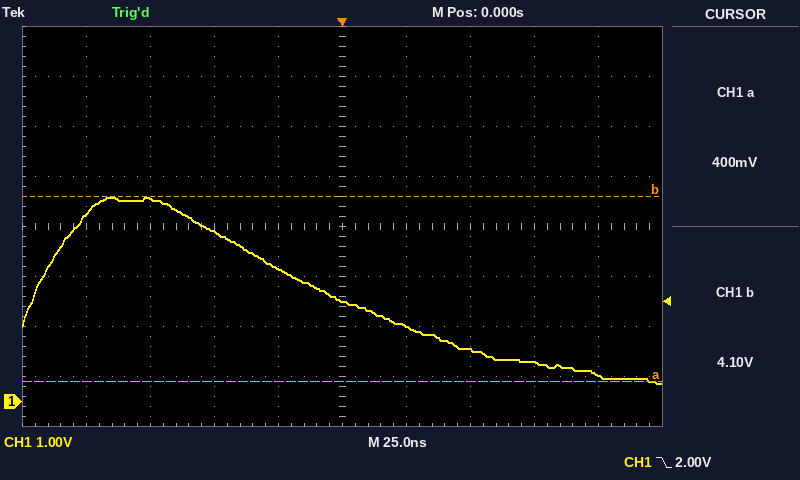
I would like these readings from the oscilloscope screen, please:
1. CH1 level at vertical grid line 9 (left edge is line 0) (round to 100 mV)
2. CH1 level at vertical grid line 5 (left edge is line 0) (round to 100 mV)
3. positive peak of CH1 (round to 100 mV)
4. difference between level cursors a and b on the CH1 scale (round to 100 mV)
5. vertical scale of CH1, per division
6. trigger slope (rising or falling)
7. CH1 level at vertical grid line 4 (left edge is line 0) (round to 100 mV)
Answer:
500 mV
2.0 V
4.1 V
3.7 V
1 V
falling
2.7 V
